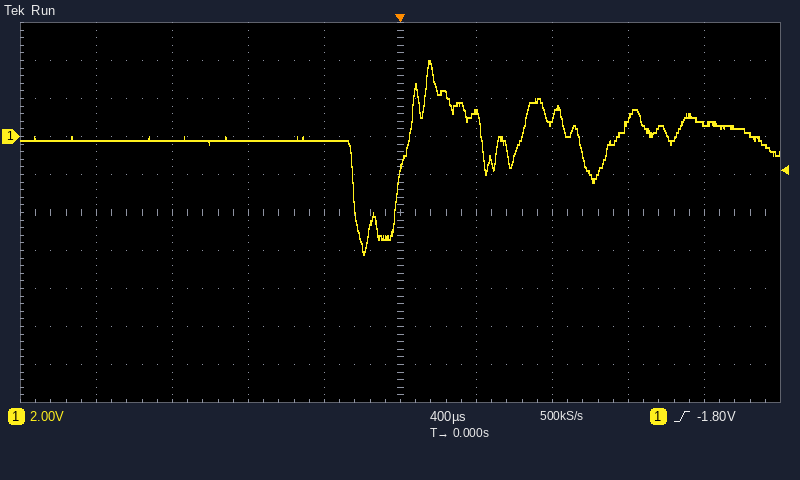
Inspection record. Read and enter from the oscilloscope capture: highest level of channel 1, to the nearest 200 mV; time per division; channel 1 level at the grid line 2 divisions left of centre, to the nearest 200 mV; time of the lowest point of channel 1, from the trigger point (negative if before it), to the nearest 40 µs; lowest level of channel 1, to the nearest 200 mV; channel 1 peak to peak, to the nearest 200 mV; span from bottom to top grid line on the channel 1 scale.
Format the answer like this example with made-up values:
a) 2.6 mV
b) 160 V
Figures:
a) 4.0 V
b) 400 µs
c) -200 mV
d) -200 µs
e) -6.2 V
f) 10.2 V
g) 20 V
